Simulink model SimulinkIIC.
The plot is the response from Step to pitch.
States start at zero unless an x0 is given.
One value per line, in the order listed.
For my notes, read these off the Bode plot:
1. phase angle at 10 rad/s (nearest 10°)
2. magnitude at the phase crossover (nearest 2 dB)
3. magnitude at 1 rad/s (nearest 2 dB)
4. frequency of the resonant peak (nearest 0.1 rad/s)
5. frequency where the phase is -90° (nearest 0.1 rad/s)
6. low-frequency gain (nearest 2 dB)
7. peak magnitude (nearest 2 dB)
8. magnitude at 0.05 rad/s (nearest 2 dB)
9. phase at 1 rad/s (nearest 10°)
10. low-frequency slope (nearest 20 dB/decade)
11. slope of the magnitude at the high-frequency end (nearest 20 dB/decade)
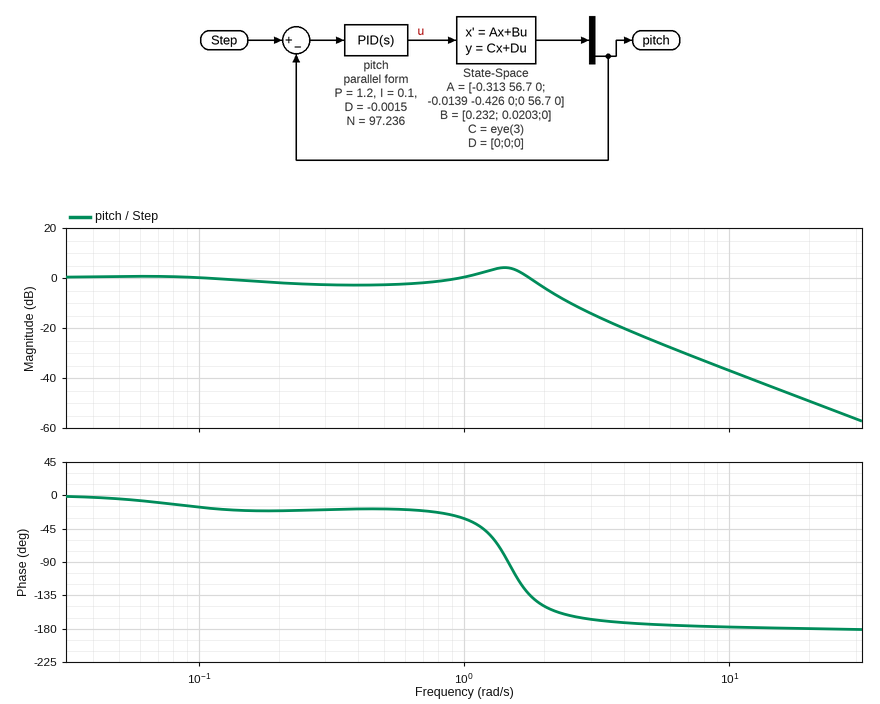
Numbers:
-180°
-50 dB
0 dB
1.4 rad/s
1.5 rad/s
0 dB
4 dB
0 dB
-30°
0 dB/decade
-40 dB/decade
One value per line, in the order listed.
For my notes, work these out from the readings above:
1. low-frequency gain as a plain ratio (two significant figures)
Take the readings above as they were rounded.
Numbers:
1.0
